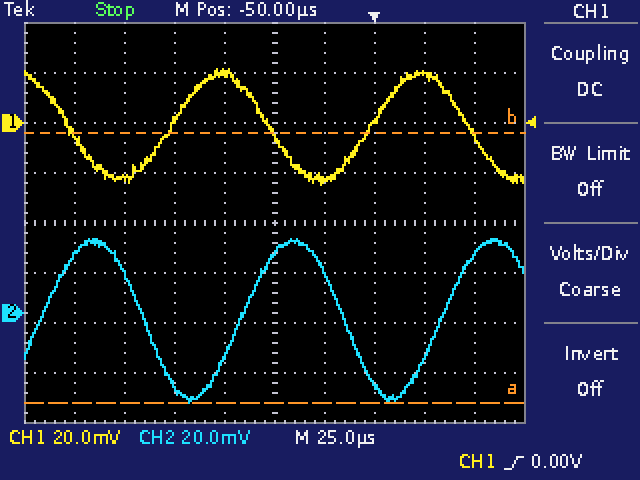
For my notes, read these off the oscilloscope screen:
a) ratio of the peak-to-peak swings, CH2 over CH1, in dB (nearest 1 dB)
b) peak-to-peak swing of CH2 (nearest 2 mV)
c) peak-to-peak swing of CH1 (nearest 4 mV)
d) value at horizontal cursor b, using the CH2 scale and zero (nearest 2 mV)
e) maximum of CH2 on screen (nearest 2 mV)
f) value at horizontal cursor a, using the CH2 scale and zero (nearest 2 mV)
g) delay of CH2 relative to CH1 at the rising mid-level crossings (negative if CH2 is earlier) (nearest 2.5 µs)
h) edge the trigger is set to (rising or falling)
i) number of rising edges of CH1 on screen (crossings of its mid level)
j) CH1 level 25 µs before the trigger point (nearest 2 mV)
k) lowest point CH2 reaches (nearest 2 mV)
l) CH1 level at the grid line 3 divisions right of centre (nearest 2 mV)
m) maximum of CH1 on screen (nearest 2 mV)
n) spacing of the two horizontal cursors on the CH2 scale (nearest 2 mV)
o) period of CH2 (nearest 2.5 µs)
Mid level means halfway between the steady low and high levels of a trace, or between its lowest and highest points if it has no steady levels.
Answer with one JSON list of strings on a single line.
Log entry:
["3 dB", "66 mV", "48 mV", "72 mV", "30 mV", "-36 mV", "+35.0 µs", "rising", "2", "-24 mV", "-36 mV", "20 mV", "22 mV", "108 mV", "100.0 µs"]
